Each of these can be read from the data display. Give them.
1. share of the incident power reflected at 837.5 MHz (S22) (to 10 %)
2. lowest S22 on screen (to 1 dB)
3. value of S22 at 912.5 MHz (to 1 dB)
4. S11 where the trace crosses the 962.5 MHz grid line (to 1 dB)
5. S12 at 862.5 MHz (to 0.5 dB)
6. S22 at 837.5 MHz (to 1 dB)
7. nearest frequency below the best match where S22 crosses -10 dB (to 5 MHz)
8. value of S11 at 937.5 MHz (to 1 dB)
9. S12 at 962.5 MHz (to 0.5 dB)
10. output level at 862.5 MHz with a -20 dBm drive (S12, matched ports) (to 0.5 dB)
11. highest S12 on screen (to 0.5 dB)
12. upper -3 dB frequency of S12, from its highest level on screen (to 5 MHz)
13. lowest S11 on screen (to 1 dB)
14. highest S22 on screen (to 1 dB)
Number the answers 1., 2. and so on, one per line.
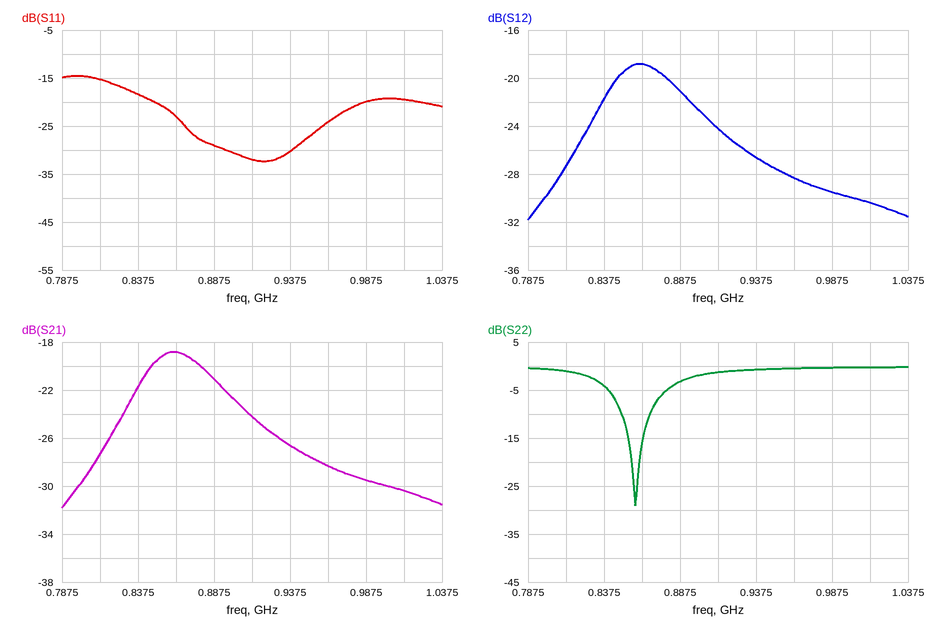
1. 40 %
2. -29 dB
3. -1 dB
4. -24 dB
5. -19.0 dB
6. -4 dB
7. 850 MHz
8. -30 dB
9. -28.5 dB
10. -39.0 dBm
11. -19.0 dB
12. 895 MHz
13. -32 dB
14. 0 dB
